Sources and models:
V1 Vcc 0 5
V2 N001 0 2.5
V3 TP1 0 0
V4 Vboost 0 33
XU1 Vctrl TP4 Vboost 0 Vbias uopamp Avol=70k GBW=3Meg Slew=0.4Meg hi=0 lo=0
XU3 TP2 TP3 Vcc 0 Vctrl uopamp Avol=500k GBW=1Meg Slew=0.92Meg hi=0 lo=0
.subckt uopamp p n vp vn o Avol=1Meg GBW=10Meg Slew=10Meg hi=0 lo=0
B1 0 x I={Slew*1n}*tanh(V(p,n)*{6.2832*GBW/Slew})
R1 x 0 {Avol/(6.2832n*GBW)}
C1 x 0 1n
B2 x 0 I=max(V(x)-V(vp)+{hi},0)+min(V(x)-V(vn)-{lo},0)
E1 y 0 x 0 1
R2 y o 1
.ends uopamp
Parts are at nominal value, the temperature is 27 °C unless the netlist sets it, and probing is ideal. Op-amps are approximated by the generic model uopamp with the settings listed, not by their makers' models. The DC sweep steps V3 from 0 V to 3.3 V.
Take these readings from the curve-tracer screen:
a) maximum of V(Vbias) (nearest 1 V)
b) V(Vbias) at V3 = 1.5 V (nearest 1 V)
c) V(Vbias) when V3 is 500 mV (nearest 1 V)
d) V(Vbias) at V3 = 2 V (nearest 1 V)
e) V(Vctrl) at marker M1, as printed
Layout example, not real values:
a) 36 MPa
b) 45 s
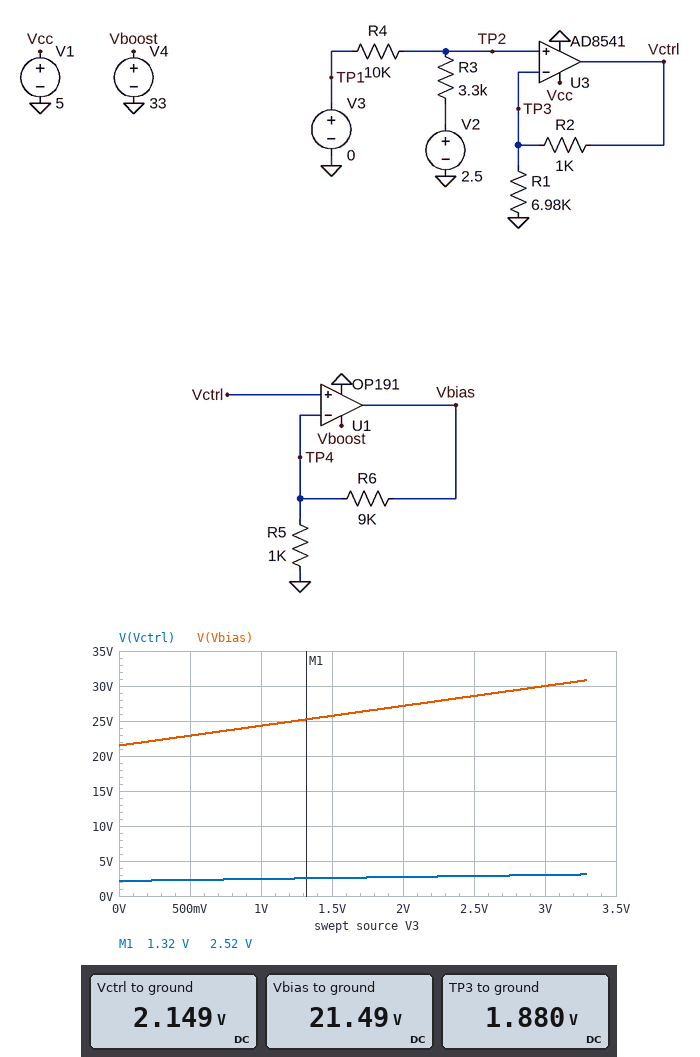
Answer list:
a) 31 V
b) 26 V
c) 23 V
d) 27 V
e) 2.52 V
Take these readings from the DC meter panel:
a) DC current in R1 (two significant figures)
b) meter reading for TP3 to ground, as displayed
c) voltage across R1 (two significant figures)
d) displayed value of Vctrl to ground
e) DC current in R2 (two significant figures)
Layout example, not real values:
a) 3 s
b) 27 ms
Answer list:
a) 270 µA
b) 1.880 V
c) 1.9 V
d) 2.149 V
e) 270 µA
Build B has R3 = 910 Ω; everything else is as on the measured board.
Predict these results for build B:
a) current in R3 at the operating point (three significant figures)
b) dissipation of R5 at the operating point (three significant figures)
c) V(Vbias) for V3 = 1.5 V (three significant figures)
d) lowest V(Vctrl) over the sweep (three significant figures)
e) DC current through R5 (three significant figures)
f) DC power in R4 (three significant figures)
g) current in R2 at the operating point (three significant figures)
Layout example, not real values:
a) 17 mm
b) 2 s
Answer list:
a) 229 µA
b) 6.86 mW
c) 27.6 V
d) 2.62 V
e) 2.62 mA
f) 525 µW
g) 328 µA
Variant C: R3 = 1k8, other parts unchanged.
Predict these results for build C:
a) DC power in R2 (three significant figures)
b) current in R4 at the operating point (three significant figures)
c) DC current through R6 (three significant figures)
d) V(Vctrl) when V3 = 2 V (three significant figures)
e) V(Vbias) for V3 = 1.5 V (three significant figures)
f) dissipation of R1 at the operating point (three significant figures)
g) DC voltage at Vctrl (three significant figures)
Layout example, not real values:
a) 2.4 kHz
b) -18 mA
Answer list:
a) 92.1 µW
b) 212 µA
c) 2.42 mA
d) 2.77 V
e) 26.8 V
f) 643 µW
g) 2.42 V
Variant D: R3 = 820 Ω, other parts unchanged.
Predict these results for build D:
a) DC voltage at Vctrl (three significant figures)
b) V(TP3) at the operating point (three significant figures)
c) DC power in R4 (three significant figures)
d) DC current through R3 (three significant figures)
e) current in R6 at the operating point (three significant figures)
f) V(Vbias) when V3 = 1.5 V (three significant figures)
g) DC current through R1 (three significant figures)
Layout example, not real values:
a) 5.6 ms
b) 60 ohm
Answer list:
a) 2.64 V
b) 2.31 V
c) 534 µW
d) 231 µA
e) 2.64 mA
f) 27.7 V
g) 331 µA
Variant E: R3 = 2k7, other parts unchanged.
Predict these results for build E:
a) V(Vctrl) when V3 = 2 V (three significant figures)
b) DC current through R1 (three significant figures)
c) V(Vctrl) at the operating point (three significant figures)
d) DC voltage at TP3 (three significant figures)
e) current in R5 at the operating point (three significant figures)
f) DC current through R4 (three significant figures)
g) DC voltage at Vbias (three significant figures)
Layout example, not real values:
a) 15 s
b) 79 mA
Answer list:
a) 2.74 V
b) 282 µA
c) 2.25 V
d) 1.97 V
e) 2.25 mA
f) 197 µA
g) 22.5 V
